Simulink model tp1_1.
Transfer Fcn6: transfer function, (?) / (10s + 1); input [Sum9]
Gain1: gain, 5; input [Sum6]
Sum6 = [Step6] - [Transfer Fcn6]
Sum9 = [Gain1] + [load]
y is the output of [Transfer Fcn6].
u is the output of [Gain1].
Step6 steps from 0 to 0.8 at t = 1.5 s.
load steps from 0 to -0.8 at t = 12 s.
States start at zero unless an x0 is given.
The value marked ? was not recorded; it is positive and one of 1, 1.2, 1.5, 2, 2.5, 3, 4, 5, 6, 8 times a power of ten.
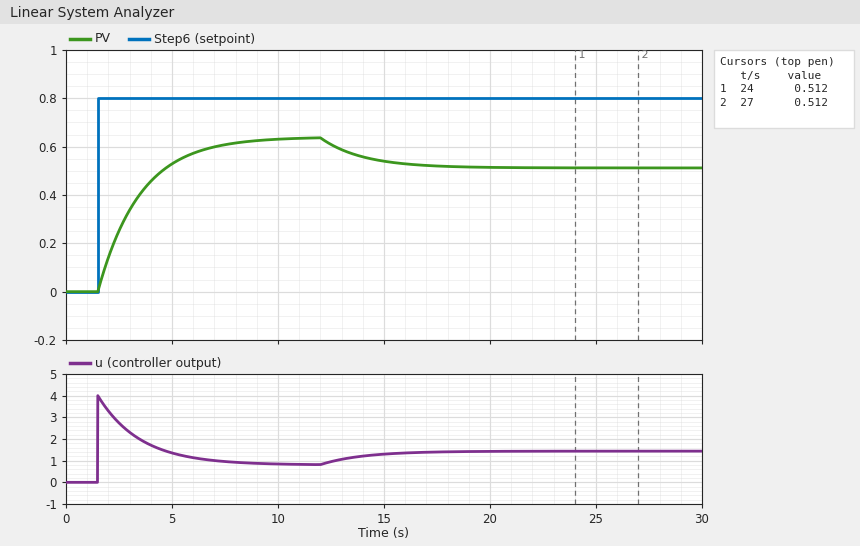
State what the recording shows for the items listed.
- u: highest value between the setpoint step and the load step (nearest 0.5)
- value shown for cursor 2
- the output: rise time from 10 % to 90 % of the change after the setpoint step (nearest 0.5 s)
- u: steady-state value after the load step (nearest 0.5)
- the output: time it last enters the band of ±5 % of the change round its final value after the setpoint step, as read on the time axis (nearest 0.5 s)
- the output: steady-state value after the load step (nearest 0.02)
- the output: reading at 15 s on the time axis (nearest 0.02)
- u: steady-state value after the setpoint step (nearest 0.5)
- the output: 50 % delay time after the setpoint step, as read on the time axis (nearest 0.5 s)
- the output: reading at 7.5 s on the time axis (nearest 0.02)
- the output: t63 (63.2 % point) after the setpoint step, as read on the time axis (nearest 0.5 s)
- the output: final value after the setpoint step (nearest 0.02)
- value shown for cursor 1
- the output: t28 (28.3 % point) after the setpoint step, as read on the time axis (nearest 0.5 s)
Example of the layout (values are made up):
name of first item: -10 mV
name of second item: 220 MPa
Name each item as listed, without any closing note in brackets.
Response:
u: highest value between the setpoint step and the load step: 4.0
value shown for cursor 2: 0.512
the output: rise time from 10 % to 90 % of the change after the setpoint step: 4.5 s
u: steady-state value after the load step: 1.5
the output: time it last enters the band of ±5 % of the change round its final value after the setpoint step, as read on the time axis: 7.5 s
the output: steady-state value after the load step: 0.52
the output: reading at 15 s on the time axis: 0.54
u: steady-state value after the setpoint step: 1.0
the output: 50 % delay time after the setpoint step, as read on the time axis: 3.0 s
the output: reading at 7.5 s on the time axis: 0.60
the output: t63 (63.2 % point) after the setpoint step, as read on the time axis: 3.5 s
the output: final value after the setpoint step: 0.64
value shown for cursor 1: 0.512
the output: t28 (28.3 % point) after the setpoint step, as read on the time axis: 2.0 s
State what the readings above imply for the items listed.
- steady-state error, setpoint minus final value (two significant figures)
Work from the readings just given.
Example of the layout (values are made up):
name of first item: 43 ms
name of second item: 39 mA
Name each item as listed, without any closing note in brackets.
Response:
steady-state error, setpoint minus final value: 0.16
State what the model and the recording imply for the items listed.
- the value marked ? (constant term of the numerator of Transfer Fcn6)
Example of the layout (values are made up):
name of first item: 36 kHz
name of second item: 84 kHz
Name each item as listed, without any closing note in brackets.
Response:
the value marked ?: 0.8
